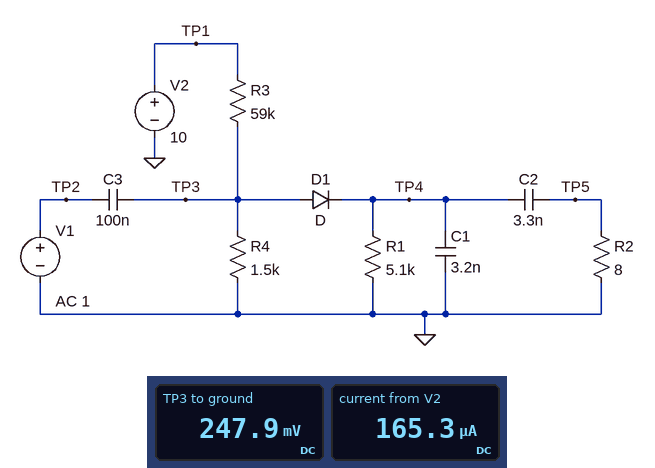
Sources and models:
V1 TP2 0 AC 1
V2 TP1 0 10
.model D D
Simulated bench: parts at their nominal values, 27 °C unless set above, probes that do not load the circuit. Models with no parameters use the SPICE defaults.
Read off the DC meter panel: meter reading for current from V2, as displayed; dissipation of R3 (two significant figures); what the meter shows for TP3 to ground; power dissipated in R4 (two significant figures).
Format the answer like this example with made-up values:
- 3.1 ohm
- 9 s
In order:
- 165.3 µA
- 1.6 mW
- 247.9 mV
- 41 µW
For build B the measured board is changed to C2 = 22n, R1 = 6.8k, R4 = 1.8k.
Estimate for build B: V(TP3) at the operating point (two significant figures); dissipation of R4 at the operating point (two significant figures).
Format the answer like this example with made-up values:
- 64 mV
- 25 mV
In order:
- 300 mV
- 49 µW
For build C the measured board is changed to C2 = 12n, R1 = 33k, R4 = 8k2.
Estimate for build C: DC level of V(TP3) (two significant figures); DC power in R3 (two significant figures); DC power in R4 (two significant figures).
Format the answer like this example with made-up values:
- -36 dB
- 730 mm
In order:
- 1.1 V
- 1.3 mW
- 150 µW
